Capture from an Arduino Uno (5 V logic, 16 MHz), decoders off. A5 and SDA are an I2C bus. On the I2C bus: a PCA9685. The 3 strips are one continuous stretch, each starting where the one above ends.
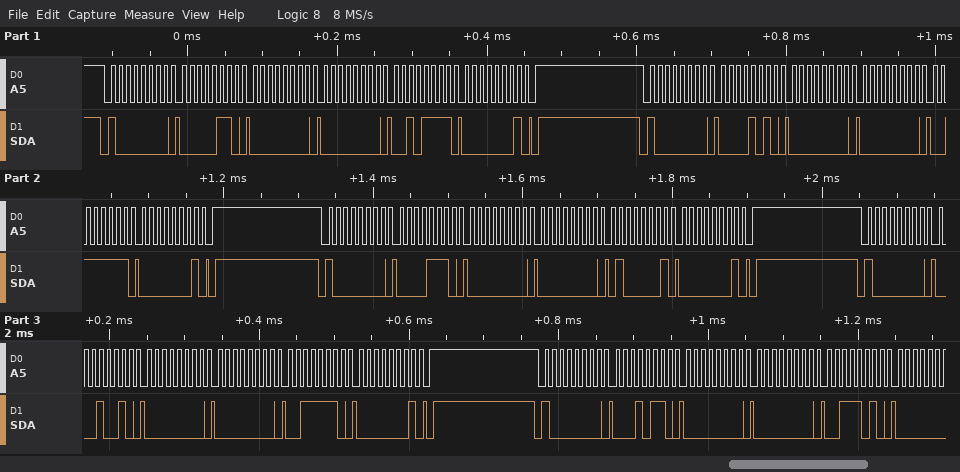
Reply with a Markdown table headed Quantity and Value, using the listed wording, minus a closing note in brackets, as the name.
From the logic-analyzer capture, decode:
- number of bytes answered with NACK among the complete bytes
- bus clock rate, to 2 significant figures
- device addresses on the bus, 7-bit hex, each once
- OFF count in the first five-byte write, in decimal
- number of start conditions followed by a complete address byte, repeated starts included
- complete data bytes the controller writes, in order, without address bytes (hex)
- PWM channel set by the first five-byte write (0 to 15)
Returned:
| Quantity | Value |
|---|---|
| number of bytes answered with NACK among the complete bytes | 0 |
| bus clock rate, to 2 significant figures | 100 kHz |
| device addresses on the bus, 7-bit hex, each once | 0x40 |
| OFF count in the first five-byte write, in decimal | 303 |
| number of start conditions followed by a complete address byte, repeated starts included | 5 |
| complete data bytes the controller writes, in order, without address bytes | 06 00 00 2F 01 0A 00 00 3F 01 0E 00 00 41 01 12 00 00 3E 01 16 00 00 3A |
| PWM channel set by the first five-byte write | 0 |
